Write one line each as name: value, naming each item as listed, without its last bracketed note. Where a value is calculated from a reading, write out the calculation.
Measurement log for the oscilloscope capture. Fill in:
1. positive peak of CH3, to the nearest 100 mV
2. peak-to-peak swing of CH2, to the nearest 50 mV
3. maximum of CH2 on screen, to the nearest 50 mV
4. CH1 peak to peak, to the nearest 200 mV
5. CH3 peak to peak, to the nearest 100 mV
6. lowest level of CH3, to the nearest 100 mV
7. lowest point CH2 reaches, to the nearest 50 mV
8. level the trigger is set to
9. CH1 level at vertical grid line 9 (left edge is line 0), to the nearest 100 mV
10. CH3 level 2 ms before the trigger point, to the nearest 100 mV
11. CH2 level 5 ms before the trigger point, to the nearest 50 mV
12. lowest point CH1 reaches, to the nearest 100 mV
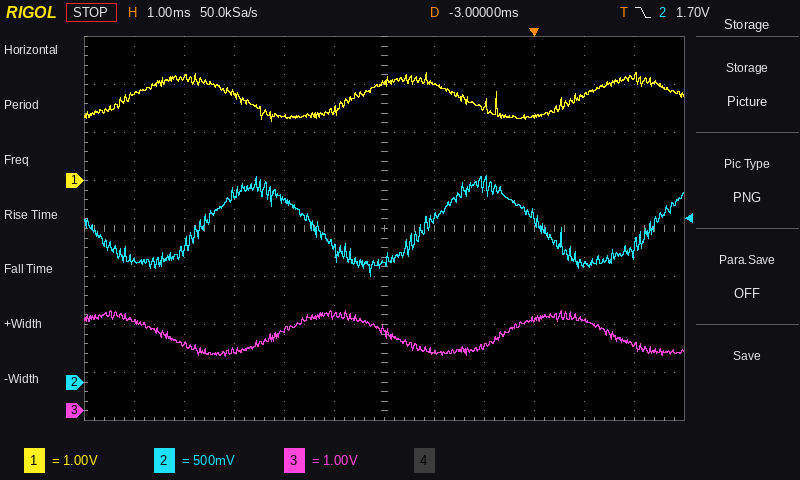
positive peak of CH3, to the nearest 100 mV: 2.1 V
peak-to-peak swing of CH2, to the nearest 50 mV: 2.15 V − (1.10 V) = 1.05 V
maximum of CH2 on screen, to the nearest 50 mV: 2.15 V
CH1 peak to peak, to the nearest 200 mV: 1.0 V
CH3 peak to peak, to the nearest 100 mV: 2.1 V − (1.1 V) = 1.0 V
lowest level of CH3, to the nearest 100 mV: 1.1 V
lowest point CH2 reaches, to the nearest 50 mV: 1.10 V
level the trigger is set to: 1.70 V
CH1 level at vertical grid line 9 (left edge is line 0), to the nearest 100 mV: 1.3 V
CH3 level 2 ms before the trigger point, to the nearest 100 mV: 1.2 V
CH2 level 5 ms before the trigger point, to the nearest 50 mV: 1.90 V
lowest point CH1 reaches, to the nearest 100 mV: 1.2 V
